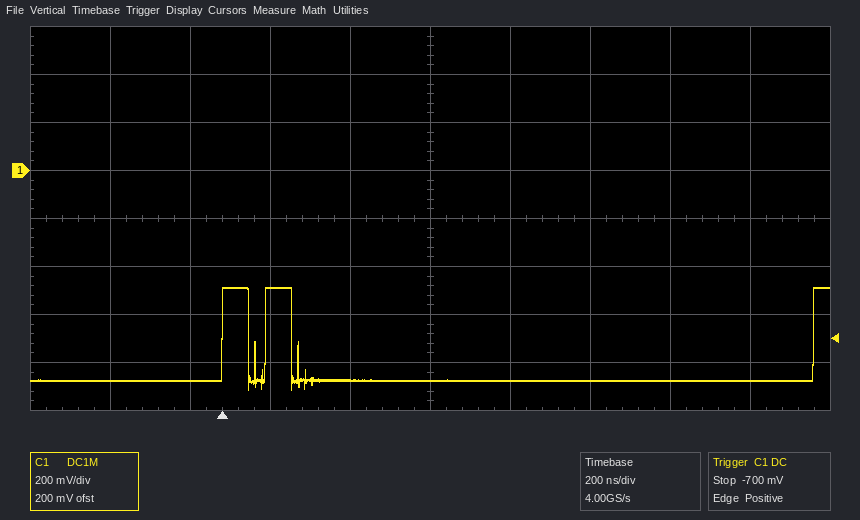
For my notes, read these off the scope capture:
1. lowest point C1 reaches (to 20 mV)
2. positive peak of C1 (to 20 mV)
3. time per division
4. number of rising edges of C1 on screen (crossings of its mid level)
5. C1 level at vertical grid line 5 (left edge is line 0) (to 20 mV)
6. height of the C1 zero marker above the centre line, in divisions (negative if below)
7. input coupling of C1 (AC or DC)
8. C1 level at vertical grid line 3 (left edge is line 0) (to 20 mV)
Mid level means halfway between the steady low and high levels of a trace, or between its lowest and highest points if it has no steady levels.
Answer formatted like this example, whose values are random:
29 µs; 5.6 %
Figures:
-920 mV; -480 mV; 200 ns; 3; -880 mV; +1.0 div; DC; -480 mV
